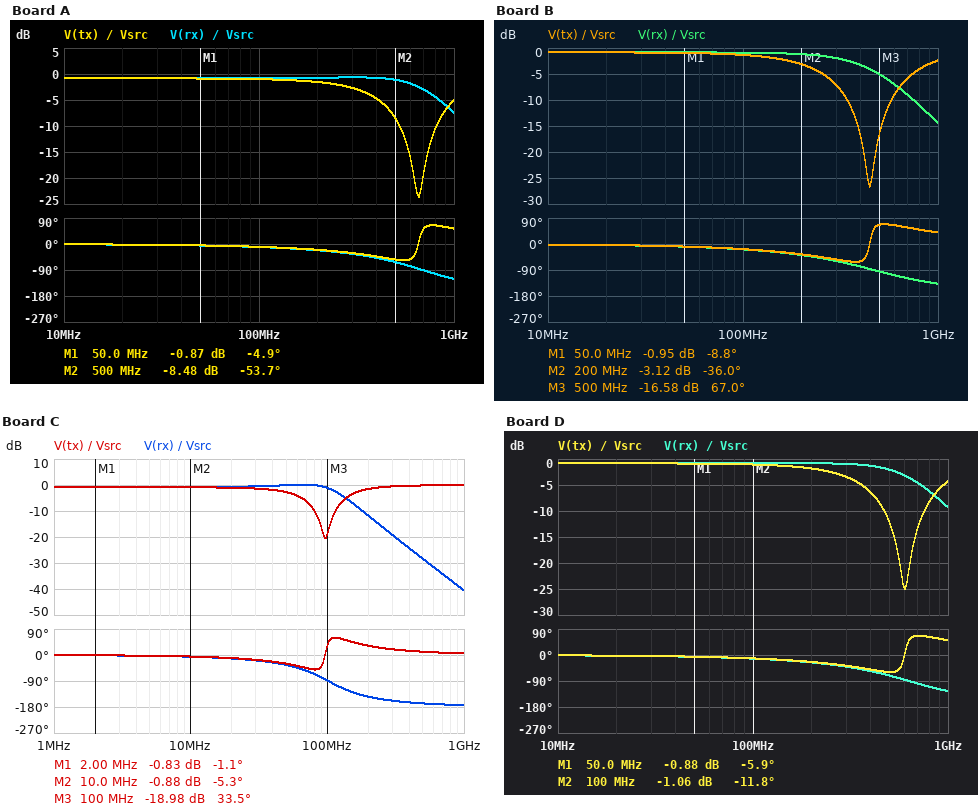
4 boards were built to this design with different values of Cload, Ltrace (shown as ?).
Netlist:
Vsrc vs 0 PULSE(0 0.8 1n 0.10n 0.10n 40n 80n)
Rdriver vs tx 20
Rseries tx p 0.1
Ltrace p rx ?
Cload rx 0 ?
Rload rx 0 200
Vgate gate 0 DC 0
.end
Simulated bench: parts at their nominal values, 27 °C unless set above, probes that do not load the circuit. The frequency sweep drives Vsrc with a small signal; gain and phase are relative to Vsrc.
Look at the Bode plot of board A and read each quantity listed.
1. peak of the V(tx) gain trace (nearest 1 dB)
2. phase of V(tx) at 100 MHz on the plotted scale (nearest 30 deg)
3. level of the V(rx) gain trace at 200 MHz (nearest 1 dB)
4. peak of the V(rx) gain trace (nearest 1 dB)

-1 dB
0 deg
-1 dB
-1 dB
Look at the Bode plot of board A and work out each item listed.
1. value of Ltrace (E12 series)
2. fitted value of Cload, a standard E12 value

3.9 nH
15 pF
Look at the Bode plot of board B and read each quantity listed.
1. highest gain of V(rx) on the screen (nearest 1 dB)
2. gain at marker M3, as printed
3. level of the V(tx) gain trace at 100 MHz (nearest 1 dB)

-1 dB
-16.58 dB
-1 dB
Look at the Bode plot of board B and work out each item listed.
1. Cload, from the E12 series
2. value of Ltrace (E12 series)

27 pF
4.7 nH
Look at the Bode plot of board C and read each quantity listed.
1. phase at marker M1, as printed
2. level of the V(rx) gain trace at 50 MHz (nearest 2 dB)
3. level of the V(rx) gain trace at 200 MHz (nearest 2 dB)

-1.1 deg
0 dB
-12 dB
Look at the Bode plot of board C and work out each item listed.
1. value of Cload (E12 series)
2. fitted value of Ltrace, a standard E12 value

82 pF
33 nH
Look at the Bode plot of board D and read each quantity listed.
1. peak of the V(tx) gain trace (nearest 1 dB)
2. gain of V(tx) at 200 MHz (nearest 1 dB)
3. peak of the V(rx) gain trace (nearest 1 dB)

-1 dB
-2 dB
-1 dB
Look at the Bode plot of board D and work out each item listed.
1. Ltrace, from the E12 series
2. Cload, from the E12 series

3.9 nH
18 pF
